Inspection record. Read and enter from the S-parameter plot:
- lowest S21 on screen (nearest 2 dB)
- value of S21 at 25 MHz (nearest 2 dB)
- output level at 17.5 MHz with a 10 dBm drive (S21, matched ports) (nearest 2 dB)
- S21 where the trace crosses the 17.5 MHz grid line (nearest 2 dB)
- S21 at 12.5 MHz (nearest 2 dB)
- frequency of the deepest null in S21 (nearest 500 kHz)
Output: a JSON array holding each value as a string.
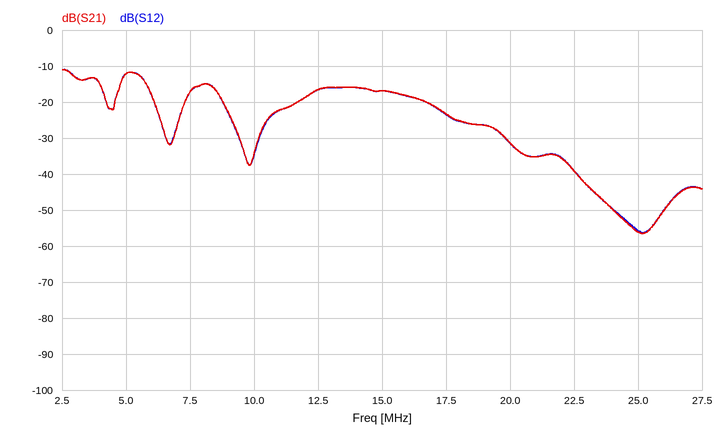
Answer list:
["-56 dB", "-56 dB", "-14 dBm", "-24 dB", "-16 dB", "25.0 MHz"]
